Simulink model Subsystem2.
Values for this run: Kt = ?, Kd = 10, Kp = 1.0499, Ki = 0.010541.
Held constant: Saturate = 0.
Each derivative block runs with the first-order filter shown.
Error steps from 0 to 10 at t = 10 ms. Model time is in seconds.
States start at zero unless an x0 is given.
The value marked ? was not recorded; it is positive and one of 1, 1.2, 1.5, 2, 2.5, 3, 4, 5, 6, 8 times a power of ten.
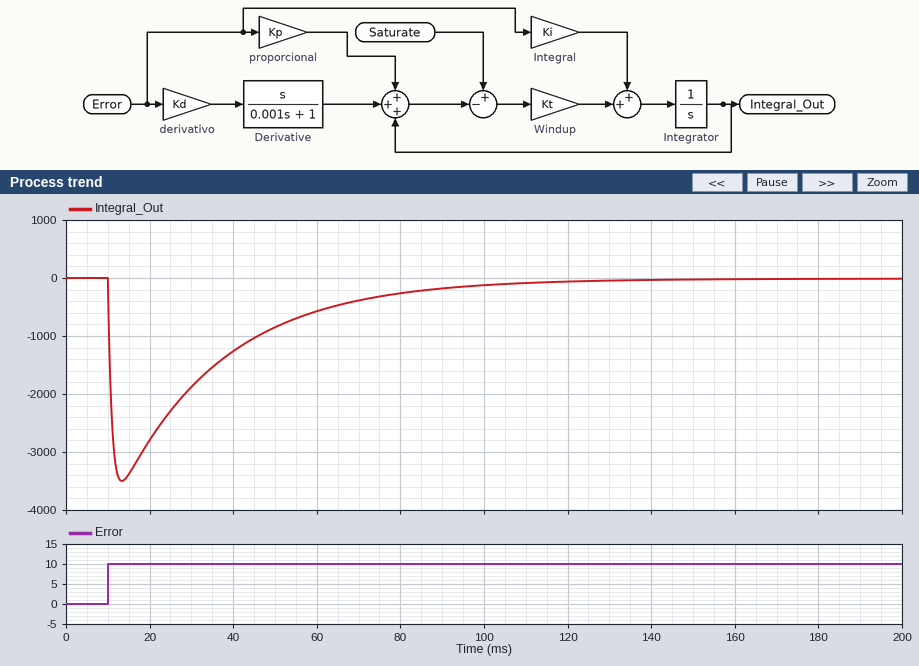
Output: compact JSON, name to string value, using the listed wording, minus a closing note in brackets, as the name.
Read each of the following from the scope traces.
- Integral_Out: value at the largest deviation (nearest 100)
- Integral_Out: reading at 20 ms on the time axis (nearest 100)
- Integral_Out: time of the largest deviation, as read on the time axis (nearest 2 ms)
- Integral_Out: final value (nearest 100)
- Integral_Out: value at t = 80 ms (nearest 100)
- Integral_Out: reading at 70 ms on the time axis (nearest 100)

{"Integral_Out: value at the largest deviation": "-3500", "Integral_Out: reading at 20 ms on the time axis": "-2800", "Integral_Out: time of the largest deviation, as read on the time axis": "14 ms", "Integral_Out: final value": "0", "Integral_Out: value at t = 80 ms": "-300", "Integral_Out: reading at 70 ms on the time axis": "-400"}
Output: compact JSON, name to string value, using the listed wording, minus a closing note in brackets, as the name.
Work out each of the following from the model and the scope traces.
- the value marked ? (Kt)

{"the value marked ?": "40"}
